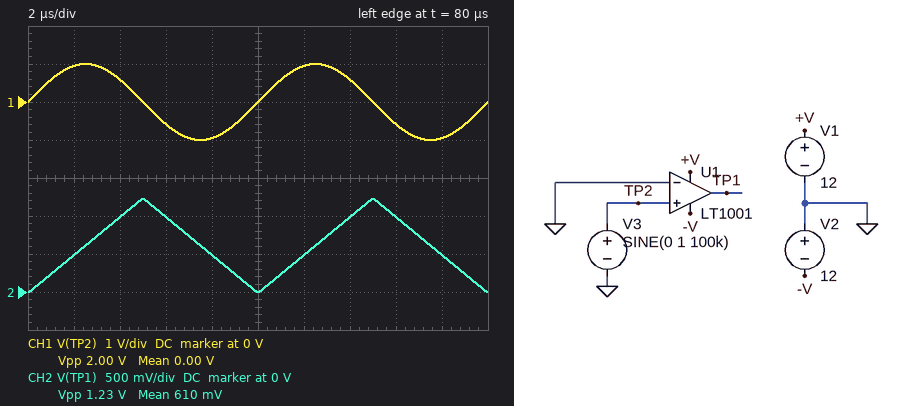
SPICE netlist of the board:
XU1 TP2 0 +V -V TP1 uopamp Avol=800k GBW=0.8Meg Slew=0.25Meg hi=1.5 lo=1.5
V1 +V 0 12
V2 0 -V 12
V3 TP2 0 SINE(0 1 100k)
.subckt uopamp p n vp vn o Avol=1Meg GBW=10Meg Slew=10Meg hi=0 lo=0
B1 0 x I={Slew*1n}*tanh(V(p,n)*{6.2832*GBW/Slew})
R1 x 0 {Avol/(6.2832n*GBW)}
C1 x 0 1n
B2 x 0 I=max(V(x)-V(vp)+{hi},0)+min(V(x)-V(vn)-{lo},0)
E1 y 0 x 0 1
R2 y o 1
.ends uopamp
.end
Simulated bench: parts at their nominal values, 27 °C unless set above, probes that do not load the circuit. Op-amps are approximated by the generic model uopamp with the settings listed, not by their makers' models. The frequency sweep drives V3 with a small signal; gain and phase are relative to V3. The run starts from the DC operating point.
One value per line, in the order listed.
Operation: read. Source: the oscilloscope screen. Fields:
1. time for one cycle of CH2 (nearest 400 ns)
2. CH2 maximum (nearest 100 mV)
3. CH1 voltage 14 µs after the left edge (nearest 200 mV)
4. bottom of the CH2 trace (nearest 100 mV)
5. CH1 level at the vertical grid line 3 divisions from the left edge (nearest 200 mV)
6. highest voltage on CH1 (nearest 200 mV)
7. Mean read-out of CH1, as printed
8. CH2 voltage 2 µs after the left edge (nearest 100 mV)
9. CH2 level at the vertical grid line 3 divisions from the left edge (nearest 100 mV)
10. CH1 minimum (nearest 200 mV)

10.0 µs
1.2 V
600 mV
0 V
-600 mV
1.0 V
0.00 V
500 mV
1.0 V
-1.0 V
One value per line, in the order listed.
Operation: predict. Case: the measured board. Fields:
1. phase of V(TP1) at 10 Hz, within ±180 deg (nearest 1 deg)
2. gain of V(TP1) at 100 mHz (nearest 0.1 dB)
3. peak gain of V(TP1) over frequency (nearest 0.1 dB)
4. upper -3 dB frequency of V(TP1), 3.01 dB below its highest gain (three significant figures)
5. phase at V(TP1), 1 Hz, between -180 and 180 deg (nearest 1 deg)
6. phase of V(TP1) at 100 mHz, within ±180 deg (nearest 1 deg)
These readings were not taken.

-84 deg
118.0 dB
118.1 dB
1.00 Hz
-45 deg
-6 deg
